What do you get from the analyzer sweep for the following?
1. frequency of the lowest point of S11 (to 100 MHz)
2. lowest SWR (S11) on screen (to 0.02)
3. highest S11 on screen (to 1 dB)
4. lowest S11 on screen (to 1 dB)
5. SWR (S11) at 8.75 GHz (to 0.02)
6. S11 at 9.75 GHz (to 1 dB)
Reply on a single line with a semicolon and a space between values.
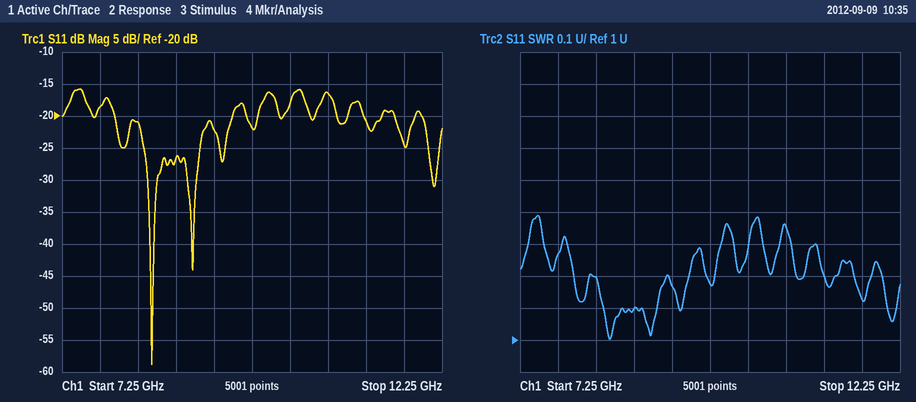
8.4 GHz; 1.00; -16 dB; -59 dB; 1.10; -22 dB
